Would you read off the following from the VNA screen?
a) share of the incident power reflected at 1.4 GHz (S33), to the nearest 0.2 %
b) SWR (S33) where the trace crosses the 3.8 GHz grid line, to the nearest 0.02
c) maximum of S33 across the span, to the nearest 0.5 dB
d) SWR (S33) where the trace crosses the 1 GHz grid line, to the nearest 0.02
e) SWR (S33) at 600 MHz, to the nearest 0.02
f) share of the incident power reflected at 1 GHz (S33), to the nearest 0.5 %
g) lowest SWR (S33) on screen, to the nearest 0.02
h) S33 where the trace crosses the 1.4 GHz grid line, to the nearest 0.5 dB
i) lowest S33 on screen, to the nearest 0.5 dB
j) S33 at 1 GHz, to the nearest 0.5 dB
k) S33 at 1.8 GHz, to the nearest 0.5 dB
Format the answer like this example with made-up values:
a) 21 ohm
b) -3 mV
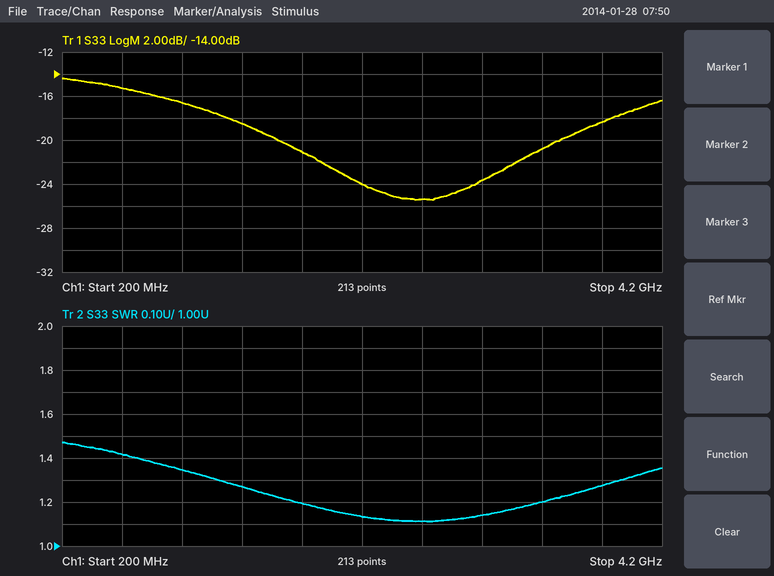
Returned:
a) 1.4 %
b) 1.28
c) -14.5 dB
d) 1.34
e) 1.42
f) 2.0 %
g) 1.12
h) -18.5 dB
i) -25.5 dB
j) -16.5 dB
k) -21.0 dB
